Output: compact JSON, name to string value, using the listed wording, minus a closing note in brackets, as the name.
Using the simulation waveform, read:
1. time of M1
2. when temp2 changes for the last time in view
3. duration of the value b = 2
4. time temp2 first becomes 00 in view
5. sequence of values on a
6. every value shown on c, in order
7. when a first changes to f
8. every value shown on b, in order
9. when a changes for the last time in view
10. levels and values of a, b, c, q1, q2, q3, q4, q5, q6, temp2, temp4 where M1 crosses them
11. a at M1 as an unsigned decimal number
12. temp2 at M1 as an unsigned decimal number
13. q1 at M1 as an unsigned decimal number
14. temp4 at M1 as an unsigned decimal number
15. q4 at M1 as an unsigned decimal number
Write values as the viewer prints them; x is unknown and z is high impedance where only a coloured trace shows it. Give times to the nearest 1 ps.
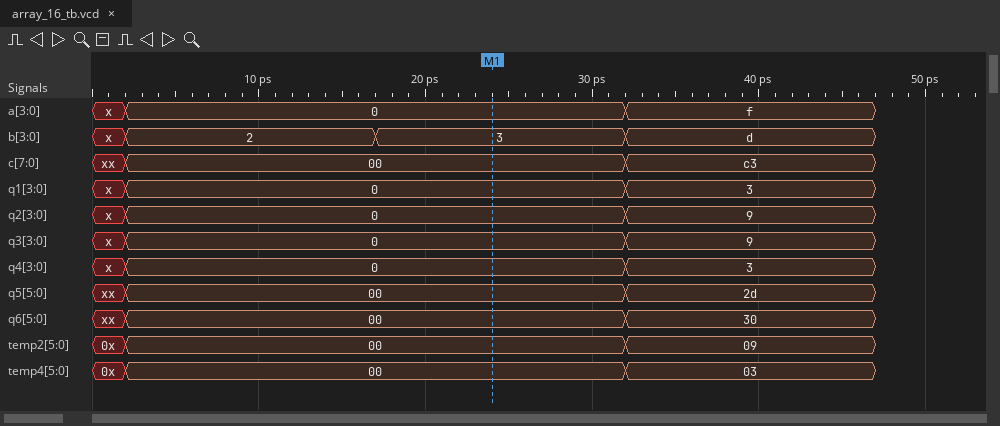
{"time of M1": "24 ps", "when temp2 changes for the last time in view": "32 ps", "duration of the value b = 2": "15 ps", "time temp2 first becomes 00 in view": "2 ps", "sequence of values on a": "x, 0, f", "every value shown on c, in order": "xx, 00, c3", "when a first changes to f": "32 ps", "every value shown on b, in order": "x, 2, 3, d", "when a changes for the last time in view": "32 ps", "levels and values of a, b, c, q1, q2, q3, q4, q5, q6, temp2, temp4 where M1 crosses them": "a=0, b=3, c=00, q1=0, q2=0, q3=0, q4=0, q5=00, q6=00, temp2=00, temp4=00", "a at M1 as an unsigned decimal number": "0", "temp2 at M1 as an unsigned decimal number": "0", "q1 at M1 as an unsigned decimal number": "0", "temp4 at M1 as an unsigned decimal number": "0", "q4 at M1 as an unsigned decimal number": "0"}
